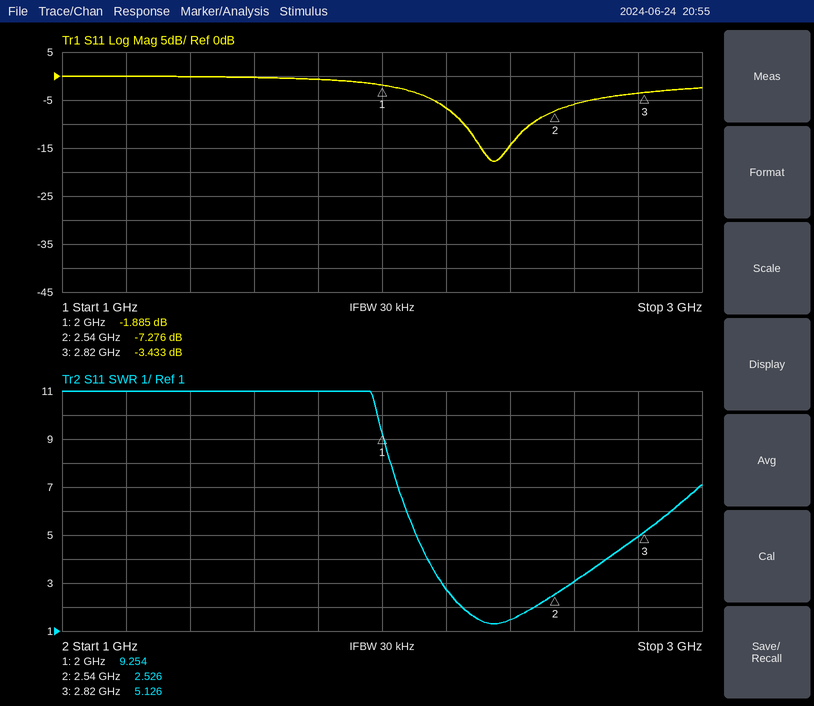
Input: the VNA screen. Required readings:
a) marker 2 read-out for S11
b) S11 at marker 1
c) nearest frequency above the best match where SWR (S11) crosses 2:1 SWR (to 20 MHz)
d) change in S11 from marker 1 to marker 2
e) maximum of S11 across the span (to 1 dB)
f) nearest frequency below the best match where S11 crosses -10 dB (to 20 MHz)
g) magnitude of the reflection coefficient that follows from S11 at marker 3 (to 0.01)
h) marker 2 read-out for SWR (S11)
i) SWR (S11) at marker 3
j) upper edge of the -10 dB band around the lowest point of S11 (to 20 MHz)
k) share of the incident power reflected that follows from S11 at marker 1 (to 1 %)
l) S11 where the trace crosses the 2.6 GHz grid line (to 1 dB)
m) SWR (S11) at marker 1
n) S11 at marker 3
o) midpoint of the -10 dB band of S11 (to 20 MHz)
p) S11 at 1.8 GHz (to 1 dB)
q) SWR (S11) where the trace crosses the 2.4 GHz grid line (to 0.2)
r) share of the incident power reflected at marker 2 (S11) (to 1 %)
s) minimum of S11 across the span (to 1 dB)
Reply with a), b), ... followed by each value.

a) -7.276 dB
b) -1.885 dB
c) 2.48 GHz
d) -5.391 dB
e) 0 dB
f) 2.26 GHz
g) 0.67
h) 2.526
i) 5.126
j) 2.46 GHz
k) 65 %
l) -6 dB
m) 9.254
n) -3.433 dB
o) 2.36 GHz
p) -1 dB
q) 1.4
r) 19 %
s) -18 dB
